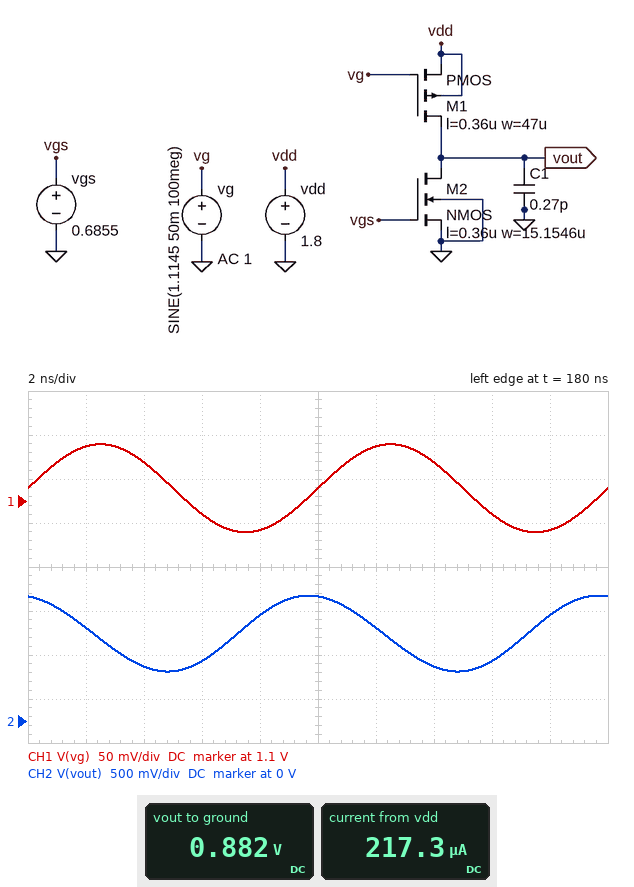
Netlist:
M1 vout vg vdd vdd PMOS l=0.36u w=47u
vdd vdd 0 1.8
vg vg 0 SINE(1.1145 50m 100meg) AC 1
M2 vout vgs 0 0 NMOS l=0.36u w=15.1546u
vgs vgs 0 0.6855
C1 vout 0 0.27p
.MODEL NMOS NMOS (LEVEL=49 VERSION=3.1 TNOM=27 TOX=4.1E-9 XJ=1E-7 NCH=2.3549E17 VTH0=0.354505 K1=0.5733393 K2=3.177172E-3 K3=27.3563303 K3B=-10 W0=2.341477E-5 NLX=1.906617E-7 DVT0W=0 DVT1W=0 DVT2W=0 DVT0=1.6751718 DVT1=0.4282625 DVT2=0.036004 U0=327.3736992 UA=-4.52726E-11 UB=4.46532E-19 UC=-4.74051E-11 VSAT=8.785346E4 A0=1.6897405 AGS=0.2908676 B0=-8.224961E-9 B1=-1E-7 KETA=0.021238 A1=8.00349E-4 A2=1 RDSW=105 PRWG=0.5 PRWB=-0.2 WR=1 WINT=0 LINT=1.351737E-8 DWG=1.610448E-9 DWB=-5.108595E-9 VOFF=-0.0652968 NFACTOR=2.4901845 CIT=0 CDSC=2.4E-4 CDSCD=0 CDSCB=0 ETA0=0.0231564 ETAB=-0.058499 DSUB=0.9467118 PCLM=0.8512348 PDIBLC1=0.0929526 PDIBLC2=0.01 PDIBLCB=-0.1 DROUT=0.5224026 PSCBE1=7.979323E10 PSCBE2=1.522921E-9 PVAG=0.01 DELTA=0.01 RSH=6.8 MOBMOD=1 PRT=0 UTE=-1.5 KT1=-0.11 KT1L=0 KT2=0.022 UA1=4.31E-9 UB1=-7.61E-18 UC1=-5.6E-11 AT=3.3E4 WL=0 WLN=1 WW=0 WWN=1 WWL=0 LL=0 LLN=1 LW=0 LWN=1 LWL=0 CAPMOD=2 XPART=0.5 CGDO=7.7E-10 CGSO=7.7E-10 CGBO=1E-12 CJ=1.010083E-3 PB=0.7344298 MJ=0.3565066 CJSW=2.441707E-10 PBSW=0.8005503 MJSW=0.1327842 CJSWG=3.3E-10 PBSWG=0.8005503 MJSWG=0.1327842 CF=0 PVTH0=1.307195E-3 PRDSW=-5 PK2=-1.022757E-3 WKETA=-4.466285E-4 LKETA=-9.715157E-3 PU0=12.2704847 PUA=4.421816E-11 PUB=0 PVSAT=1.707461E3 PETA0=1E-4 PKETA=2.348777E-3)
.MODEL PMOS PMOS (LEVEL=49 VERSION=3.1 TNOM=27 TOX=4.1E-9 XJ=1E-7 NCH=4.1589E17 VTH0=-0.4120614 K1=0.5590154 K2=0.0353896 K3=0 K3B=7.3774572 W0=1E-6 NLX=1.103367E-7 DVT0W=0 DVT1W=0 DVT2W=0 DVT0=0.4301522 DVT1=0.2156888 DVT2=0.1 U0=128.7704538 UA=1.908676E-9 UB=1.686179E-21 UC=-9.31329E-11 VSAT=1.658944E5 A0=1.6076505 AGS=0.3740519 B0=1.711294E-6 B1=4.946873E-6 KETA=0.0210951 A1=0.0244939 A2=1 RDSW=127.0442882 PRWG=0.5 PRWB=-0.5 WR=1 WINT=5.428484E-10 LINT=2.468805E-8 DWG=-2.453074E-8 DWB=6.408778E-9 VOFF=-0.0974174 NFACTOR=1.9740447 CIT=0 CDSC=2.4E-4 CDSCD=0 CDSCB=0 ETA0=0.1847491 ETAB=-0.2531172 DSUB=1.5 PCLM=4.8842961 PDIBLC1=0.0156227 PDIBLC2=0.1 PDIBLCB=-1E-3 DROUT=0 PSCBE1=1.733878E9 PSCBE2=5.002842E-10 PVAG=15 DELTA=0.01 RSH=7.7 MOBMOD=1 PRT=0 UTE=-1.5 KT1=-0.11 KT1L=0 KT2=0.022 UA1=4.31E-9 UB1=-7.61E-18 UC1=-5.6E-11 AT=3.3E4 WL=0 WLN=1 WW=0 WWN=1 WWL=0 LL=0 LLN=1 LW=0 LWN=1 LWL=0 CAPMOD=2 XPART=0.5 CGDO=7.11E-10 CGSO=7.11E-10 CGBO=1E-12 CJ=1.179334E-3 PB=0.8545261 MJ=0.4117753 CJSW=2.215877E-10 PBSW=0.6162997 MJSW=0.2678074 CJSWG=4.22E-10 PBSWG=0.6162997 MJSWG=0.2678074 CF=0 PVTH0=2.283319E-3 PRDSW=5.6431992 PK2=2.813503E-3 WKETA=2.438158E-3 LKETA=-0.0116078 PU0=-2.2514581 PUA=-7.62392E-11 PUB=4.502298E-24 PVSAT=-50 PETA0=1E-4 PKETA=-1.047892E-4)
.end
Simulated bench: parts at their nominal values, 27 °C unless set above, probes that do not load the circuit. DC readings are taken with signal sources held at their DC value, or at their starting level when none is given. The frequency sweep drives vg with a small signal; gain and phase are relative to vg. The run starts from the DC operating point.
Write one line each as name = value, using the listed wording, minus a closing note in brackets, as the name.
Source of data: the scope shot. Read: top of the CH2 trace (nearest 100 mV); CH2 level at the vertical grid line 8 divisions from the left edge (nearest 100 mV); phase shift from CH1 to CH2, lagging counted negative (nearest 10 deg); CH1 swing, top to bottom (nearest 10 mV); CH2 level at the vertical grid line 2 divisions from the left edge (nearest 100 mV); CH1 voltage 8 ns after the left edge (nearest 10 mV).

top of the CH2 trace = 1.4 V
CH2 level at the vertical grid line 8 divisions from the left edge = 700 mV
phase shift from CH1 to CH2, lagging counted negative = 100 deg
CH1 swing, top to bottom = 100 mV
CH2 level at the vertical grid line 2 divisions from the left edge = 600 mV
CH1 voltage 8 ns after the left edge = 1.07 V
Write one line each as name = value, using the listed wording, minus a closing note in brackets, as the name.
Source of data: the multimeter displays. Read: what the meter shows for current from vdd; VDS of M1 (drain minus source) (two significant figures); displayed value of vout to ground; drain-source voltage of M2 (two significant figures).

what the meter shows for current from vdd = 217.3 µA
VDS of M1 (drain minus source) = -920 mV
displayed value of vout to ground = 0.882 V
drain-source voltage of M2 = 880 mV
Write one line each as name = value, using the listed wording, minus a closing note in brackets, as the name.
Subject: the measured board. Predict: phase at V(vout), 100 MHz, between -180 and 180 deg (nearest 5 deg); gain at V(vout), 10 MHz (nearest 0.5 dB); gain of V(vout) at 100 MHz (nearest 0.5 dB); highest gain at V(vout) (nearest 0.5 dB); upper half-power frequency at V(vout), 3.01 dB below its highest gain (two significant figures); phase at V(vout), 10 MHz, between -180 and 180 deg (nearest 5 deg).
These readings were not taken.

phase at V(vout), 100 MHz, between -180 and 180 deg = 100 deg
gain at V(vout), 10 MHz = 32.5 dB
gain of V(vout) at 100 MHz = 19.0 dB
highest gain at V(vout) = 33.5 dB
upper half-power frequency at V(vout), 3.01 dB below its highest gain = 19 MHz
phase at V(vout), 10 MHz, between -180 and 180 deg = 150 deg
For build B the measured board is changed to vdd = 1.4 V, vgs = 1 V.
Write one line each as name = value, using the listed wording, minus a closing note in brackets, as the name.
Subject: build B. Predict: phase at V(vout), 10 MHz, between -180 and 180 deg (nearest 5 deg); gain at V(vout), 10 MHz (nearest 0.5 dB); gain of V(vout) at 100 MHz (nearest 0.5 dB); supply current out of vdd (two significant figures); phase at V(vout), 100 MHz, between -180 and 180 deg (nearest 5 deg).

phase at V(vout), 10 MHz, between -180 and 180 deg = 145 deg
gain at V(vout), 10 MHz = -63.0 dB
gain of V(vout) at 100 MHz = -48.0 dB
supply current out of vdd = 130 nA
phase at V(vout), 100 MHz, between -180 and 180 deg = 95 deg
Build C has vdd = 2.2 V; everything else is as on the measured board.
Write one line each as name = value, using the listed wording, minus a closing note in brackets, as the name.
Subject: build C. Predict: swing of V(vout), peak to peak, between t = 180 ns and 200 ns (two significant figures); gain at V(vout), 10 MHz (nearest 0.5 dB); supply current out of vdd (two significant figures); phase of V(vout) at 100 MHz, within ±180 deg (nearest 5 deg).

swing of V(vout), peak to peak, between t = 180 ns and 200 ns = 7.1 mV
gain at V(vout), 10 MHz = -23.0 dB
supply current out of vdd = 240 µA
phase of V(vout) at 100 MHz, within ±180 deg = 165 deg
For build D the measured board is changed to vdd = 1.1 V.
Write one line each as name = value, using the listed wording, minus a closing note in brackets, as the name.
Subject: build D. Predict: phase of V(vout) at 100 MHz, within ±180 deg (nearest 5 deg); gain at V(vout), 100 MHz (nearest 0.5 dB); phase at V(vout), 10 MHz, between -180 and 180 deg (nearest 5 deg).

phase of V(vout) at 100 MHz, within ±180 deg = 85 deg
gain at V(vout), 100 MHz = -40.5 dB
phase at V(vout), 10 MHz, between -180 and 180 deg = 90 deg
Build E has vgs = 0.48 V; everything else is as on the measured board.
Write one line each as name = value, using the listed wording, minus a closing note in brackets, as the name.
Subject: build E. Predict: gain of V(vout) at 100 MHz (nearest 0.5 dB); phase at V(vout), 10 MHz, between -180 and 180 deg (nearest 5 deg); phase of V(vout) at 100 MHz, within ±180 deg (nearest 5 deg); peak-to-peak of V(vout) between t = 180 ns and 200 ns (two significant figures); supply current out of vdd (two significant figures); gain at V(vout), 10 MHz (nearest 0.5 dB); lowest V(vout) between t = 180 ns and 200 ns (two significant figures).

gain of V(vout) at 100 MHz = -29.0 dB
phase at V(vout), 10 MHz, between -180 and 180 deg = 170 deg
phase of V(vout) at 100 MHz, within ±180 deg = 115 deg
peak-to-peak of V(vout) between t = 180 ns and 200 ns = 3.8 mV
supply current out of vdd = 8.1 µA
gain at V(vout), 10 MHz = -34.0 dB
lowest V(vout) between t = 180 ns and 200 ns = 1.8 V
